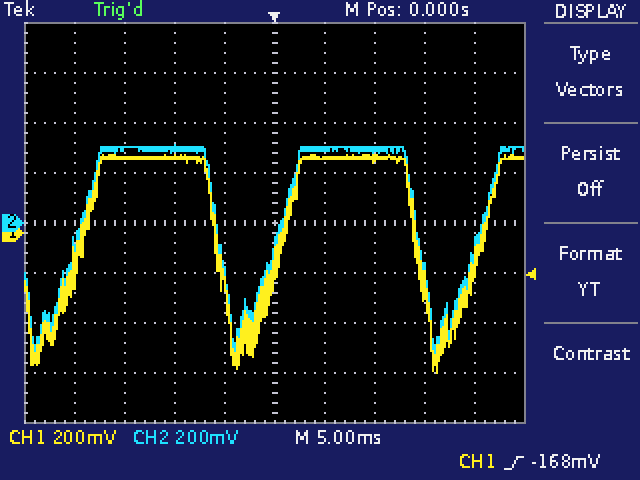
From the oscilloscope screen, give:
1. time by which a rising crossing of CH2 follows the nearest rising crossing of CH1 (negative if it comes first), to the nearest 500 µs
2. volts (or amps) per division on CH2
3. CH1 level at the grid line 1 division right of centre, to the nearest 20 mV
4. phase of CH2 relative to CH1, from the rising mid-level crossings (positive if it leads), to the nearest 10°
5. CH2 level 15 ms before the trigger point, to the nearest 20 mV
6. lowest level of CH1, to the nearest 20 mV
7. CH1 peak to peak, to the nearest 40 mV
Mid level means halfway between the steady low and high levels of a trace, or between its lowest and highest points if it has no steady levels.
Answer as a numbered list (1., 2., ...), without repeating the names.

1. 0.0 ms
2. 200 mV
3. 300 mV
4. 0°
5. 300 mV
6. -560 mV
7. 880 mV
